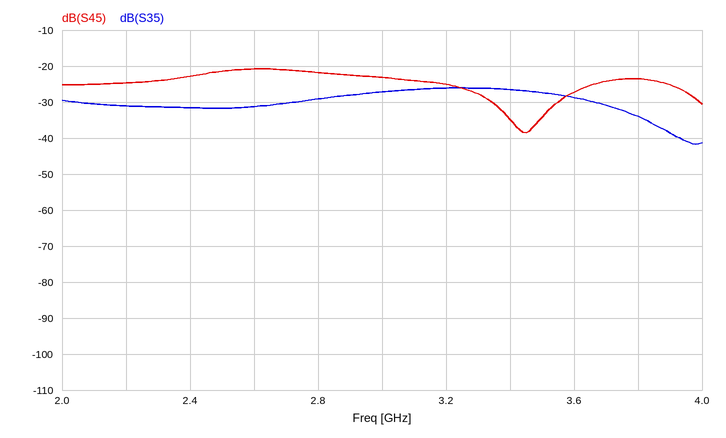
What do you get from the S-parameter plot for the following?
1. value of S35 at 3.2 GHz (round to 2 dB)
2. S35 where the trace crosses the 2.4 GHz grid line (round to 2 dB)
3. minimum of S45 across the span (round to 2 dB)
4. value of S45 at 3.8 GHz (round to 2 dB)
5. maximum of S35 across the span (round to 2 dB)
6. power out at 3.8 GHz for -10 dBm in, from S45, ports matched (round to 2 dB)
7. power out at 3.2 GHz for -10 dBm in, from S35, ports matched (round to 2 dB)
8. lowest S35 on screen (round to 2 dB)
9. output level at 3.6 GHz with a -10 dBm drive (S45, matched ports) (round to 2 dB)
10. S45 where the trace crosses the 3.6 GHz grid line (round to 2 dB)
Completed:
-26 dB
-32 dB
-38 dB
-24 dB
-26 dB
-34 dBm
-36 dBm
-42 dB
-38 dBm
-28 dB
